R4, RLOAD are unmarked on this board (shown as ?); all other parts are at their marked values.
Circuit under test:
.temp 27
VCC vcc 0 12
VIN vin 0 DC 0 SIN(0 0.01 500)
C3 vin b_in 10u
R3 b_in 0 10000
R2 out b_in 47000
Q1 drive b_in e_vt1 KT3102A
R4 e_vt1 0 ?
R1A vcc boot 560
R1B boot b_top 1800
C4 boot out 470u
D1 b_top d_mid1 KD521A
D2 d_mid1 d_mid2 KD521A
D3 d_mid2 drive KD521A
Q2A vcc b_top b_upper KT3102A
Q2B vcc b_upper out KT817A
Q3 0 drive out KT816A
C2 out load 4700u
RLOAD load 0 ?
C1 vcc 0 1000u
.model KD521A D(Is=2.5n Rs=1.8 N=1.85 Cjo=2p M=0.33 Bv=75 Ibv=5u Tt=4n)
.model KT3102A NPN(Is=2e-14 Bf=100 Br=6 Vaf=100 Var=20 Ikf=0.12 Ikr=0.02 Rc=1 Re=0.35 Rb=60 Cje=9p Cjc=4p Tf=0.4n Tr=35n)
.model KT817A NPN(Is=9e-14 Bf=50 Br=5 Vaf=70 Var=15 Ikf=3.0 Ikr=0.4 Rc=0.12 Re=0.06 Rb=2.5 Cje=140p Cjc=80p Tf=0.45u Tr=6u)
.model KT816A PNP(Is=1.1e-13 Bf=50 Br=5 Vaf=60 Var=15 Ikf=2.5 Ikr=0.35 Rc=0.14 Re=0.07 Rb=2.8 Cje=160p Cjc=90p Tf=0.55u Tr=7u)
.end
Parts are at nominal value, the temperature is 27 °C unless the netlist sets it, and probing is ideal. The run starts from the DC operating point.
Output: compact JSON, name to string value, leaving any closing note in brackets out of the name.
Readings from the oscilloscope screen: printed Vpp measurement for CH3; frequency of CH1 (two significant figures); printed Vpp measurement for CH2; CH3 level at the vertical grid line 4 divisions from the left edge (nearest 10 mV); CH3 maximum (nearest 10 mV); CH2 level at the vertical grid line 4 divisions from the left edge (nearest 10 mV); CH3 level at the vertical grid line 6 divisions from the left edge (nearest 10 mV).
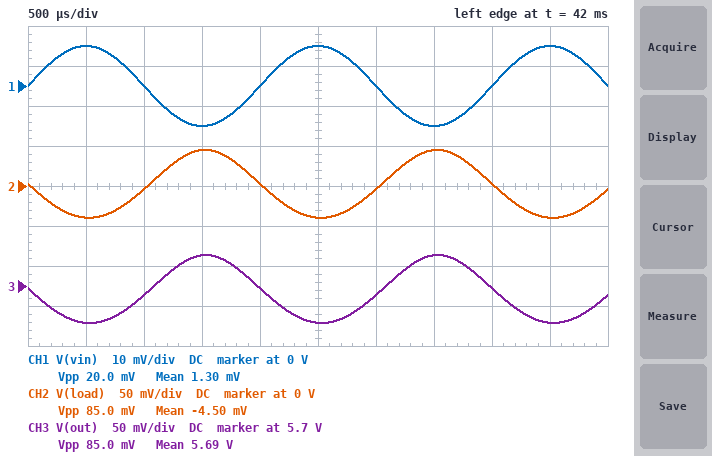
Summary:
{"printed Vpp measurement for CH3": "85.0 mV", "frequency of CH1": "500 Hz", "printed Vpp measurement for CH2": "85.0 mV", "CH3 level at the vertical grid line 4 divisions from the left edge": "5.70 V", "CH3 maximum": "5.74 V", "CH2 level at the vertical grid line 4 divisions from the left edge": "0 V", "CH3 level at the vertical grid line 6 divisions from the left edge": "5.69 V"}
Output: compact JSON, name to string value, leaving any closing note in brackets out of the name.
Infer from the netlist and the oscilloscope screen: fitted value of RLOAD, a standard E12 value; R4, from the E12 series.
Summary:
{"fitted value of RLOAD, a standard E12 value": "3.3 Ω", "R4, from the E12 series": "47 Ω"}
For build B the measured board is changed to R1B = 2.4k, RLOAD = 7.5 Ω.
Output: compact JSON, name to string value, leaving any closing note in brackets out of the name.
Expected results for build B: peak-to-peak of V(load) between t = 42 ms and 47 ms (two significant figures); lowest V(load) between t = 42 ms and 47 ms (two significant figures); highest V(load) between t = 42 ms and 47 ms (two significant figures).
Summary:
{"peak-to-peak of V(load) between t = 42 ms and 47 ms": "190 mV", "lowest V(load) between t = 42 ms and 47 ms": "-86 mV", "highest V(load) between t = 42 ms and 47 ms": "100 mV"}
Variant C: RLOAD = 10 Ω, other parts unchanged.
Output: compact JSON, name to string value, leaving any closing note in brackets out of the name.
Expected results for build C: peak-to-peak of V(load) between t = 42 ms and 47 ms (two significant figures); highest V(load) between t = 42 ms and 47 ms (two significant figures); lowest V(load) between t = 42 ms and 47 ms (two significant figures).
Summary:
{"peak-to-peak of V(load) between t = 42 ms and 47 ms": "250 mV", "highest V(load) between t = 42 ms and 47 ms": "130 mV", "lowest V(load) between t = 42 ms and 47 ms": "-120 mV"}
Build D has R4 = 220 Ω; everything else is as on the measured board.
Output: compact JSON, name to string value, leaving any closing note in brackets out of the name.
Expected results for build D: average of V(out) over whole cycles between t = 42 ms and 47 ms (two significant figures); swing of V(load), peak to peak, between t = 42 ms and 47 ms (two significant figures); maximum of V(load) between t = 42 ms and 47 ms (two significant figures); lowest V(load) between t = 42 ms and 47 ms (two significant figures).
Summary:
{"average of V(out) over whole cycles between t = 42 ms and 47 ms": "6.9 V", "swing of V(load), peak to peak, between t = 42 ms and 47 ms": "21 mV", "maximum of V(load) between t = 42 ms and 47 ms": "11 mV", "lowest V(load) between t = 42 ms and 47 ms": "-10 mV"}
